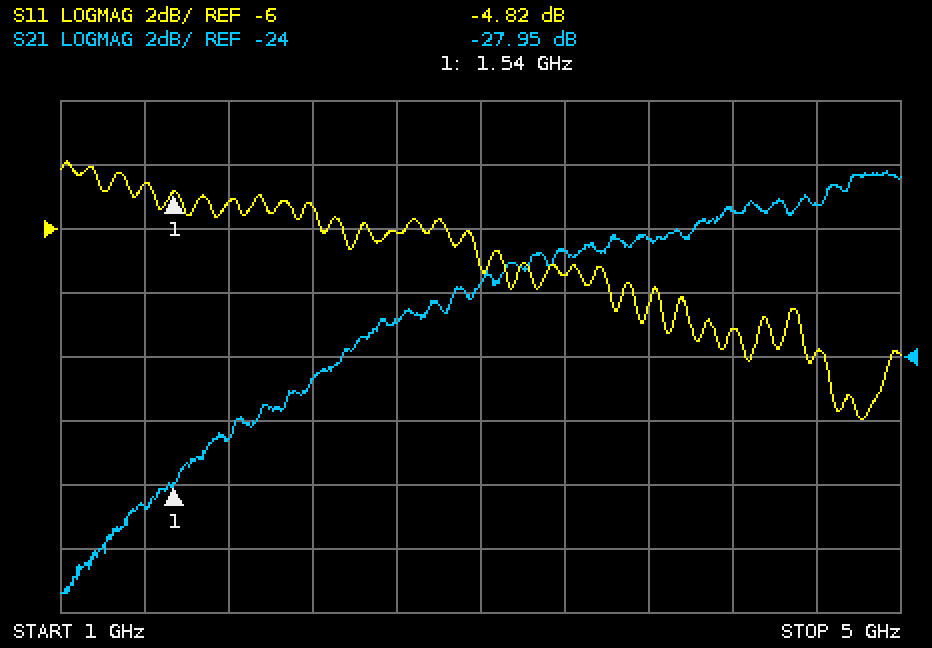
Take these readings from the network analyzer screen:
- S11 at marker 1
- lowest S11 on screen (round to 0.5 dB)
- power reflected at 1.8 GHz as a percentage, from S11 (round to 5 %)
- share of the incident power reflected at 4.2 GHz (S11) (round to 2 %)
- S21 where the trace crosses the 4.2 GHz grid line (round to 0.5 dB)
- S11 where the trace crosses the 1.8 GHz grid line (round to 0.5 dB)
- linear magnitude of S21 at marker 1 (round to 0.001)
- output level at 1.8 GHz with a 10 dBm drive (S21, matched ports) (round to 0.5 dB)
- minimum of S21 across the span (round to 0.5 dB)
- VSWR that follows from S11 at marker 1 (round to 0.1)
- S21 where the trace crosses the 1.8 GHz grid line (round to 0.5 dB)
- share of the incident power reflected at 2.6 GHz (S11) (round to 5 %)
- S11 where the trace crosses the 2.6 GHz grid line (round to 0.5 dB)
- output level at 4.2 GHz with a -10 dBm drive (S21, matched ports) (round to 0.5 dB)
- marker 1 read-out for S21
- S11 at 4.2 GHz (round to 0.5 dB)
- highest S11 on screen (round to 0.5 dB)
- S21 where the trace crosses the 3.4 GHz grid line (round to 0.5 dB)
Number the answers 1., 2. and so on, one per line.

1. -4.82 dB
2. -12.0 dB
3. 30 %
4. 12 %
5. -19.5 dB
6. -5.0 dB
7. 0.040
8. -16.5 dBm
9. -31.5 dB
10. 3.7
11. -26.5 dB
12. 25 %
13. -6.0 dB
14. -29.5 dBm
15. -27.95 dB
16. -9.0 dB
17. -4.0 dB
18. -20.5 dB
